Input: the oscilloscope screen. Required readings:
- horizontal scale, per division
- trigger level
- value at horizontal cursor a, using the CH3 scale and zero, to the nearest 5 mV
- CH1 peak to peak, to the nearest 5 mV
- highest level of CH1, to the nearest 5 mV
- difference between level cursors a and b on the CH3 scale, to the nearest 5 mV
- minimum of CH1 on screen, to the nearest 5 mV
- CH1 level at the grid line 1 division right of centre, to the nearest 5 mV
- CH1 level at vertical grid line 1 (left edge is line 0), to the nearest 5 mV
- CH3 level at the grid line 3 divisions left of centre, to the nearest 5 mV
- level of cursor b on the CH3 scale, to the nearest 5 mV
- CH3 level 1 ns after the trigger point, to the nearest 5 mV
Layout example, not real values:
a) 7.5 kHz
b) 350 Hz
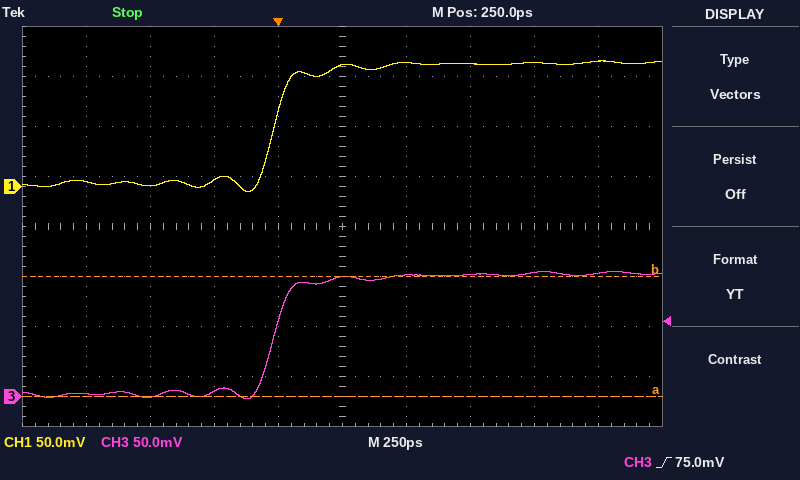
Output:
a) 250 ps
b) 75.0 mV
c) 0 mV
d) 130 mV
e) 125 mV
f) 120 mV
g) -5 mV
h) 125 mV
i) 5 mV
j) 0 mV
k) 120 mV
l) 125 mV
